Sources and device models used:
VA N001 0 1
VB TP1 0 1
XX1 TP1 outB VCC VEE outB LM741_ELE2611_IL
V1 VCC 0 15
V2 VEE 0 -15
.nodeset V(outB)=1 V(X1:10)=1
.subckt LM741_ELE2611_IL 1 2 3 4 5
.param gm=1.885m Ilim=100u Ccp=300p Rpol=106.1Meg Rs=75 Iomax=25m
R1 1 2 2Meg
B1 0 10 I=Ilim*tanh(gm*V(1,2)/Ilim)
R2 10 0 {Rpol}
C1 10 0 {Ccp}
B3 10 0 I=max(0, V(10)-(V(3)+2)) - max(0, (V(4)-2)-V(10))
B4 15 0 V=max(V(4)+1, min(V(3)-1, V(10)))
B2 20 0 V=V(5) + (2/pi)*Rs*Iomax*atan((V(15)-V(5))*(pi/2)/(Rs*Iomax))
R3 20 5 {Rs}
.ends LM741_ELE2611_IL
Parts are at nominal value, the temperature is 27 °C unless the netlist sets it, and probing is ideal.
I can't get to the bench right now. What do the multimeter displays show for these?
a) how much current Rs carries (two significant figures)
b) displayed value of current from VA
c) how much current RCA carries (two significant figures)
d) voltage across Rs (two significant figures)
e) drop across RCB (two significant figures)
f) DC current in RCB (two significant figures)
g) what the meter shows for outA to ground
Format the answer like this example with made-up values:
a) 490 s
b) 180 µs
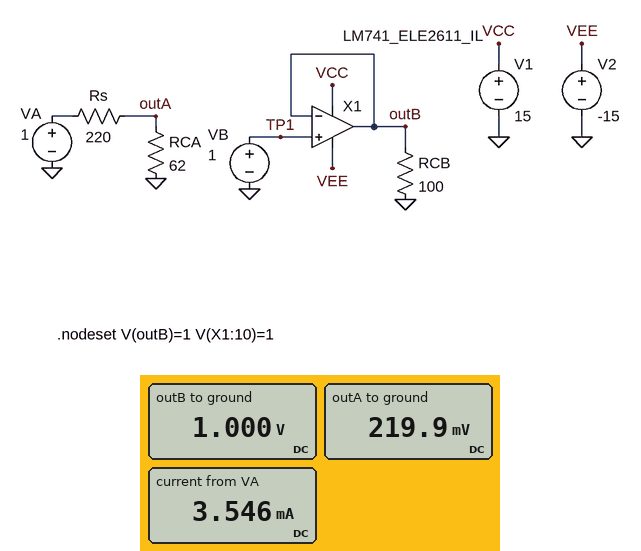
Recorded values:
a) 3.5 mA
b) 3.546 mA
c) 3.5 mA
d) 780 mV
e) 1.0 V
f) 10 mA
g) 219.9 mV
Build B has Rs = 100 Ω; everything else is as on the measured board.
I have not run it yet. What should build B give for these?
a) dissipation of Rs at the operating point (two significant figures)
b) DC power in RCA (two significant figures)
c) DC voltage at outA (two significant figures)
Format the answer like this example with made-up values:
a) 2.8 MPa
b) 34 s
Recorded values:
a) 3.8 mW
b) 2.4 mW
c) 380 mV
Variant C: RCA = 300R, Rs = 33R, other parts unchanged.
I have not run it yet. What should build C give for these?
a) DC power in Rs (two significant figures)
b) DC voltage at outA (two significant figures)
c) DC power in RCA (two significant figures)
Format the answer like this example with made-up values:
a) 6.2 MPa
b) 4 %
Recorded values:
a) 300 µW
b) 900 mV
c) 2.7 mW
